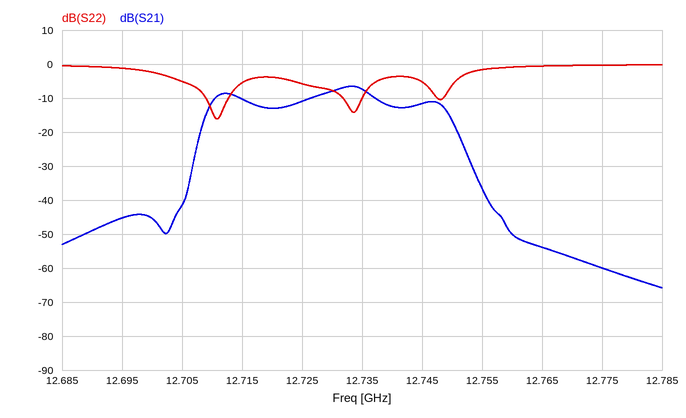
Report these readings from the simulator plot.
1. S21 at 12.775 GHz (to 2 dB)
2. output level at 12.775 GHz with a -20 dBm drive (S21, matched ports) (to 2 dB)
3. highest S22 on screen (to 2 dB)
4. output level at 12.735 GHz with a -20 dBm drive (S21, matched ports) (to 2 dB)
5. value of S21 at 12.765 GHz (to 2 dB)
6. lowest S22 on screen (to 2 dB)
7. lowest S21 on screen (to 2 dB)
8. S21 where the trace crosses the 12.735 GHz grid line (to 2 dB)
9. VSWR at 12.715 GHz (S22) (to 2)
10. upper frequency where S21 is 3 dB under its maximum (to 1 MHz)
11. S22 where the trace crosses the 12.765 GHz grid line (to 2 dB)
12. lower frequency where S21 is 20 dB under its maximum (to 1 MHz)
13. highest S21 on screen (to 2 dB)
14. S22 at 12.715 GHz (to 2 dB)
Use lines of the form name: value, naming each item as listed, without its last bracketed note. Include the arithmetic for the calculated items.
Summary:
S21 at 12.775 GHz: -60 dB
output level at 12.775 GHz with a -20 dBm drive (S21, matched ports): -20 dBm + (-60 dB) = -80 dBm
highest S22 on screen: 0 dB
output level at 12.735 GHz with a -20 dBm drive (S21, matched ports): -20 dBm + (-8 dB) = -28 dBm
value of S21 at 12.765 GHz: -54 dB
lowest S22 on screen: -16 dB
lowest S21 on screen: -66 dB
S21 where the trace crosses the 12.735 GHz grid line: -8 dB
VSWR at 12.715 GHz (S22): |Γ| = 10^(-6/20) = 0.5012; VSWR = (1 + 0.5012)/(1 − 0.5012) ≈ 3.01, so 4 to the nearest 2
upper frequency where S21 is 3 dB under its maximum: 12.737 GHz
S22 where the trace crosses the 12.765 GHz grid line: 0 dB
lower frequency where S21 is 20 dB under its maximum: 12.707 GHz
highest S21 on screen: -6 dB
S22 at 12.715 GHz: -6 dB
